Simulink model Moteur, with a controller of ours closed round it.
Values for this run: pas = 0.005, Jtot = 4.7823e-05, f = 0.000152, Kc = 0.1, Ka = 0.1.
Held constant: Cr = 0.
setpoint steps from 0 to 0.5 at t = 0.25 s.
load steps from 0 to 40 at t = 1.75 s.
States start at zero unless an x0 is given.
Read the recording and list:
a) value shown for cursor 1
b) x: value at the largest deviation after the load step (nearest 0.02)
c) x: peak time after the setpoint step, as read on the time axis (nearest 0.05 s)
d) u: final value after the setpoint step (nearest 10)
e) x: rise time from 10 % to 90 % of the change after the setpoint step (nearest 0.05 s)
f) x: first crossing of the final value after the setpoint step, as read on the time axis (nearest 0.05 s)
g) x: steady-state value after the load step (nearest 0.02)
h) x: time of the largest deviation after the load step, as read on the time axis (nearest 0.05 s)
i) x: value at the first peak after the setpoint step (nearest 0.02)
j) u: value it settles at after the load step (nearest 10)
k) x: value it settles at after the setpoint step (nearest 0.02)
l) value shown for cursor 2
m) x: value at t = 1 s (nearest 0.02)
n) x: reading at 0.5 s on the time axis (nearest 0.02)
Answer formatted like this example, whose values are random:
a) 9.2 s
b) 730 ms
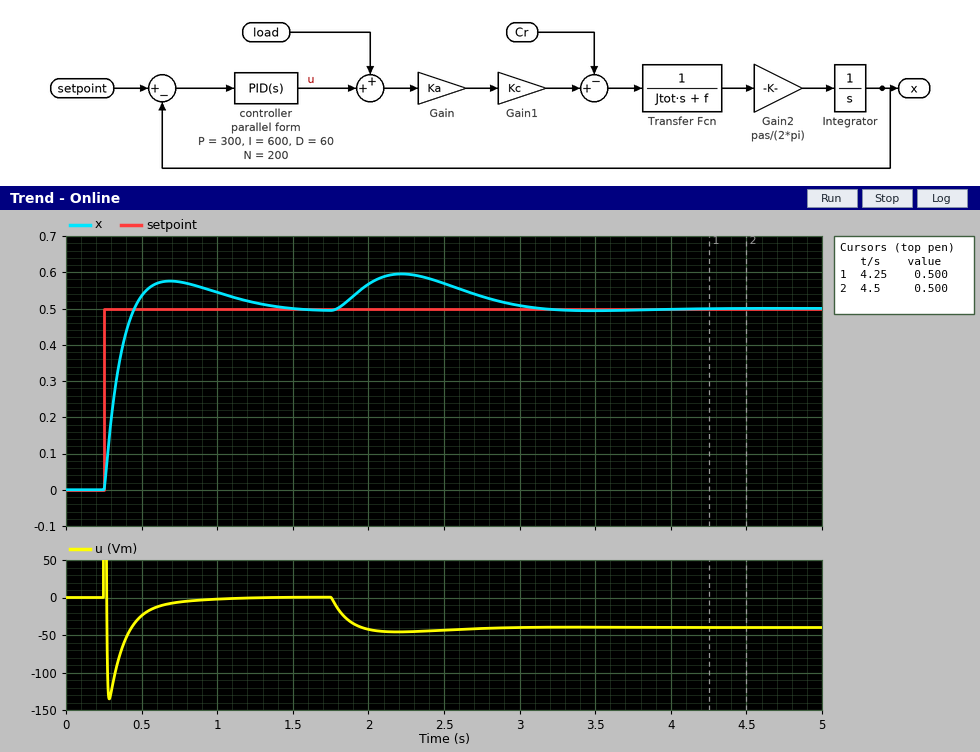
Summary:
a) 0.500
b) 0.60
c) 0.70 s
d) 0
e) 0.15 s
f) 0.45 s
g) 0.50
h) 2.20 s
i) 0.58
j) -40
k) 0.50
l) 0.500
m) 0.54
n) 0.54
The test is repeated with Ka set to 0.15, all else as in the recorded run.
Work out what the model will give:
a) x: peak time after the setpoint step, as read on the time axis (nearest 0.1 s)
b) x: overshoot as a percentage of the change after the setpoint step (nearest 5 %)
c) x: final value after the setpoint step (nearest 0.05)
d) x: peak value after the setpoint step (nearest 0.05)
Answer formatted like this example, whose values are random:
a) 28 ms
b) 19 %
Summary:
a) 0.6 s
b) 10 %
c) 0.50
d) 0.55
